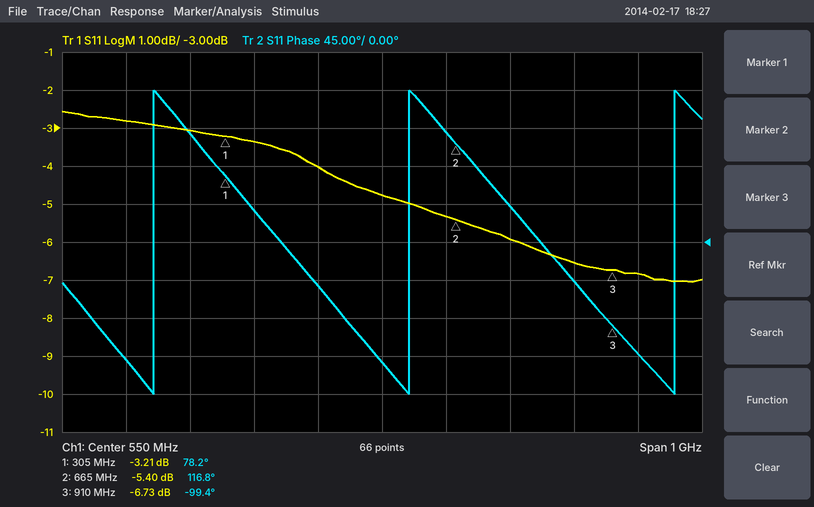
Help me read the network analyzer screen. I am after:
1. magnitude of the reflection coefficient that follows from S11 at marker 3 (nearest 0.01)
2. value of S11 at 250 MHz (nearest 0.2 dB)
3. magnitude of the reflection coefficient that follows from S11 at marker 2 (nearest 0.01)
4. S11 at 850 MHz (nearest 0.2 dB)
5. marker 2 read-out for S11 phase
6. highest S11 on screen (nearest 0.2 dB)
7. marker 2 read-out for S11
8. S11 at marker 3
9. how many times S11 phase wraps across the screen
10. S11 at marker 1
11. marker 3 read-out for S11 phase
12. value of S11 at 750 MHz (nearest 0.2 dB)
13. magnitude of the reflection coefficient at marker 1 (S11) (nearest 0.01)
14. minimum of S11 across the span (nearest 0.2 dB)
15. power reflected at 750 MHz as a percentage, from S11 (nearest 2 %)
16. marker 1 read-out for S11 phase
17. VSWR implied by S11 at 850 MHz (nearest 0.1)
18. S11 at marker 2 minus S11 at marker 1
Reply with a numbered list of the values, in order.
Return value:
1. 0.46
2. -3.0 dB
3. 0.54
4. -6.6 dB
5. 116.8°
6. -2.6 dB
7. -5.40 dB
8. -6.73 dB
9. 3
10. -3.21 dB
11. -99.4°
12. -6.0 dB
13. 0.69
14. -7.0 dB
15. 26 %
16. 78.2°
17. 2.8
18. -2.19 dB
